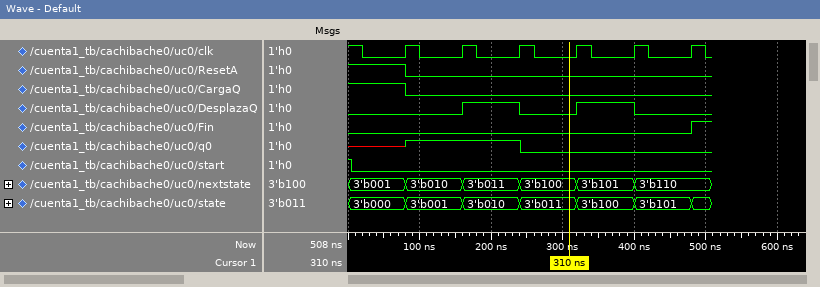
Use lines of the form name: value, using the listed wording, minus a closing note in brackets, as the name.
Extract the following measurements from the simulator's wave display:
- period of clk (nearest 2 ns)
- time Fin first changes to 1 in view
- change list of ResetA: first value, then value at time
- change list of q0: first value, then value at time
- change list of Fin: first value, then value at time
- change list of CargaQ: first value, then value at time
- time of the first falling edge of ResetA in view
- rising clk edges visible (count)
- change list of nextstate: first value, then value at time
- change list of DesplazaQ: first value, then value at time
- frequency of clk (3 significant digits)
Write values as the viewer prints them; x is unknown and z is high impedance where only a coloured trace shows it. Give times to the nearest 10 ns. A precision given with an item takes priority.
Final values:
period of clk: 80 ns
time Fin first changes to 1 in view: 480 ns
change list of ResetA: first value, then value at time: 1, 0 at 80 ns
change list of q0: first value, then value at time: x, 1 at 80 ns, 0 at 240 ns
change list of Fin: first value, then value at time: 0, 1 at 480 ns
change list of CargaQ: first value, then value at time: 1, 0 at 80 ns
time of the first falling edge of ResetA in view: 80 ns
rising clk edges visible: 6
change list of nextstate: first value, then value at time: 3'b001, 3'b010 at 80 ns, 3'b011 at 160 ns, 3'b100 at 240 ns, 3'b101 at 320 ns, 3'b110 at 400 ns
change list of DesplazaQ: first value, then value at time: 0, 1 at 160 ns, 0 at 240 ns, 1 at 320 ns, 0 at 400 ns
frequency of clk: 12.5 MHz
